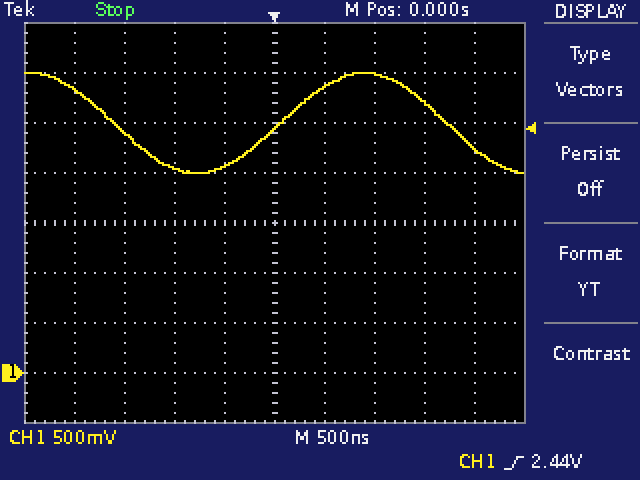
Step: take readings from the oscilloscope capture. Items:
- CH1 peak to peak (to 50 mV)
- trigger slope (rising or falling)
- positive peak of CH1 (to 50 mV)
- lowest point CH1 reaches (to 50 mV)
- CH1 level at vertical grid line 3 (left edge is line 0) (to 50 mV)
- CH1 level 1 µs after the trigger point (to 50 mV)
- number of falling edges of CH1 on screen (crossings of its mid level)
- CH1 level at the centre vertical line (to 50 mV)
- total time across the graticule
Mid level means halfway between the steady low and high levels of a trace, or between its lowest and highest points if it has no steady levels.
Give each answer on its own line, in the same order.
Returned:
1.00 V
rising
3.00 V
2.00 V
2.05 V
3.00 V
2
2.45 V
5 µs
